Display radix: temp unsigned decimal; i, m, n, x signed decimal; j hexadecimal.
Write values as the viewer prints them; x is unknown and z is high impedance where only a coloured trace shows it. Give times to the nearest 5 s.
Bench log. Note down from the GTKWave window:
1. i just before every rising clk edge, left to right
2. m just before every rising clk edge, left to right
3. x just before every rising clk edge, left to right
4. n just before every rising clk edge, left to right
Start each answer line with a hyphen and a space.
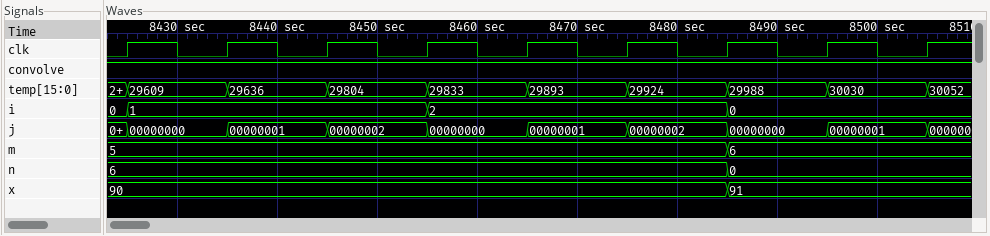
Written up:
- 0, 1, 1, 1, 2, 2, 2, 0, 0
- 5, 5, 5, 5, 5, 5, 5, 6, 6
- 90, 90, 90, 90, 90, 90, 90, 91, 91
- 6, 6, 6, 6, 6, 6, 6, 0, 0
